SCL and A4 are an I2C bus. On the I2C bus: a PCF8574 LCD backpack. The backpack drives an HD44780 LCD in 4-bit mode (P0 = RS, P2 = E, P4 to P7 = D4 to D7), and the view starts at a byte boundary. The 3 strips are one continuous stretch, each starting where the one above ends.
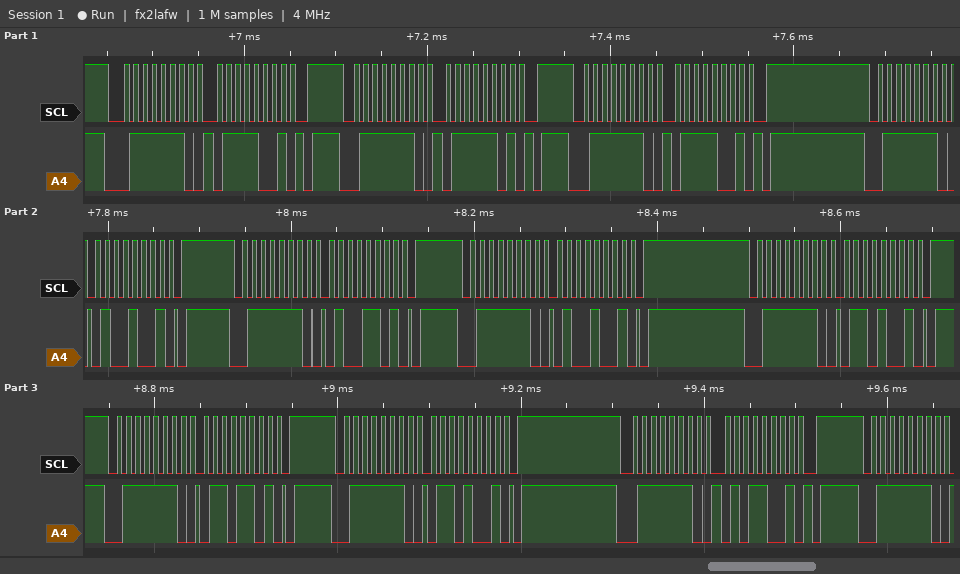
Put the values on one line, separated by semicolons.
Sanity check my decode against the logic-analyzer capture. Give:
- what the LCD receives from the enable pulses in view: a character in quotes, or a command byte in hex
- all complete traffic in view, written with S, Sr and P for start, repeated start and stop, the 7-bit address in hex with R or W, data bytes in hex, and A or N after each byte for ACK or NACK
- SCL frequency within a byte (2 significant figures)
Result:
't'; S 3FW A 79 A P S 3FW A 7D A P S 3FW A 79 A P S 3FW A 49 A P S 3FW A 4D A P S 3FW A 49 A P S 3FW A 69 A P S 3FW A 6D A P S 3FW A 69 A P S 3FW A 59 A P S 3FW A; 100 kHz
